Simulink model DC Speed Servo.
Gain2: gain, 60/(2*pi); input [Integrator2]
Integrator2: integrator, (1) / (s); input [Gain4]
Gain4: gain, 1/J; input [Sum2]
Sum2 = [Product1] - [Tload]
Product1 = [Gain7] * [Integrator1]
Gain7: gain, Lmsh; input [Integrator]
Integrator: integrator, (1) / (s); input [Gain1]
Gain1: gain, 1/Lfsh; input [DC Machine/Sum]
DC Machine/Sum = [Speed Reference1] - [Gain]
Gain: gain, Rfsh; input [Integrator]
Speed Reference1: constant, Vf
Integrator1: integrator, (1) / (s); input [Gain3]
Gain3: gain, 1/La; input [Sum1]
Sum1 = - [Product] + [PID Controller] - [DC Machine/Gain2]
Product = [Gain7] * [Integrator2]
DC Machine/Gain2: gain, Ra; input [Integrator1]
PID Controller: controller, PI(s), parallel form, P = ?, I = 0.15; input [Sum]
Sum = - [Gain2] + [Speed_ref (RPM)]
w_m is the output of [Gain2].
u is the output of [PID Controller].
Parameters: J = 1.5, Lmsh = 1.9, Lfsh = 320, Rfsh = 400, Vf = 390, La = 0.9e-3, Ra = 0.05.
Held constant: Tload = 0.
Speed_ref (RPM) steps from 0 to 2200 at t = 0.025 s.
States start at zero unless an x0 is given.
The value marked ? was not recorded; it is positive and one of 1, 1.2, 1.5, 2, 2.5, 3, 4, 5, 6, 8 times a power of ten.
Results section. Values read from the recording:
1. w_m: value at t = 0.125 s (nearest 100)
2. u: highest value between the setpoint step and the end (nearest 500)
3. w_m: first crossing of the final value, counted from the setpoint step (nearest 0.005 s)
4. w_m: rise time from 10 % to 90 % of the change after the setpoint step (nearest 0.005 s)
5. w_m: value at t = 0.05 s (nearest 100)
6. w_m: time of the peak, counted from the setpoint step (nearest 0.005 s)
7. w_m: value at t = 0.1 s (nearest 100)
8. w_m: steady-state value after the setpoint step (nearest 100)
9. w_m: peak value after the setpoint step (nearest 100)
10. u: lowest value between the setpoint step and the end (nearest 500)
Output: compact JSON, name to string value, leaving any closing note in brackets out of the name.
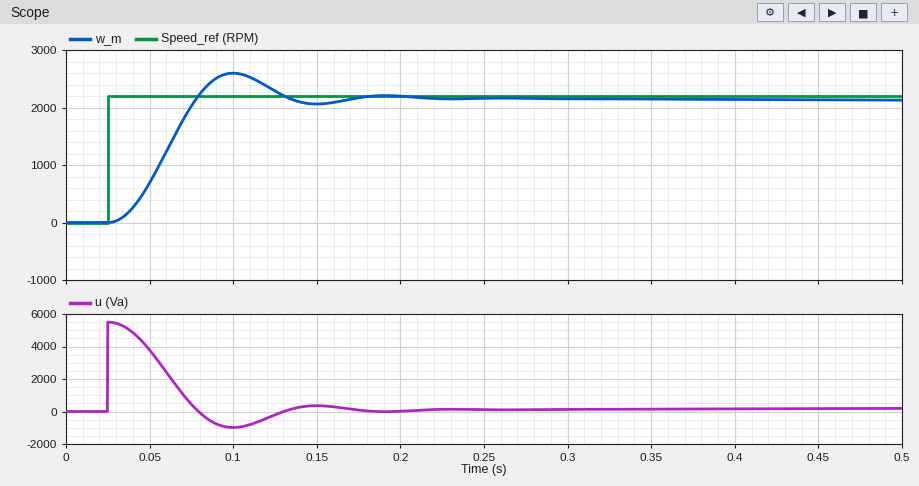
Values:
{"w_m: value at t = 0.125 s": "2300", "u: highest value between the setpoint step and the end": "5500", "w_m: first crossing of the final value, counted from the setpoint step": "0.050 s", "w_m: rise time from 10 % to 90 % of the change after the setpoint step": "0.035 s", "w_m: value at t = 0.05 s": "700", "w_m: time of the peak, counted from the setpoint step": "0.075 s", "w_m: value at t = 0.1 s": "2600", "w_m: steady-state value after the setpoint step": "2100", "w_m: peak value after the setpoint step": "2600", "u: lowest value between the setpoint step and the end": "-1000"}
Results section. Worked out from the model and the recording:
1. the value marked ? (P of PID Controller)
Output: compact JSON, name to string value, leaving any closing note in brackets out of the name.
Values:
{"the value marked ?": "2.5"}
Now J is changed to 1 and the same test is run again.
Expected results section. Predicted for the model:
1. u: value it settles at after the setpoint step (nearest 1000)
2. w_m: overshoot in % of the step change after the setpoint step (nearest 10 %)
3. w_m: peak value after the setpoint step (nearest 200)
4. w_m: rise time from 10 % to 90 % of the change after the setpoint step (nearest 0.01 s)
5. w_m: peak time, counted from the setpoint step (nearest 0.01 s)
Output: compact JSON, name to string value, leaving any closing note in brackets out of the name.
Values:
{"u: value it settles at after the setpoint step": "0", "w_m: overshoot in % of the step change after the setpoint step": "30 %", "w_m: peak value after the setpoint step": "2800", "w_m: rise time from 10 % to 90 % of the change after the setpoint step": "0.03 s", "w_m: peak time, counted from the setpoint step": "0.06 s"}
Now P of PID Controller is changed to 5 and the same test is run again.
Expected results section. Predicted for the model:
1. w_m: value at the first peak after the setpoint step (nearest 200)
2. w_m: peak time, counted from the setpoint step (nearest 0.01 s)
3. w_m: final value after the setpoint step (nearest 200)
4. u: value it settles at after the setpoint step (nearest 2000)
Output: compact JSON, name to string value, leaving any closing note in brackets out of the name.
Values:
{"w_m: value at the first peak after the setpoint step": "2800", "w_m: peak time, counted from the setpoint step": "0.05 s", "w_m: final value after the setpoint step": "2200", "u: value it settles at after the setpoint step": "0"}
